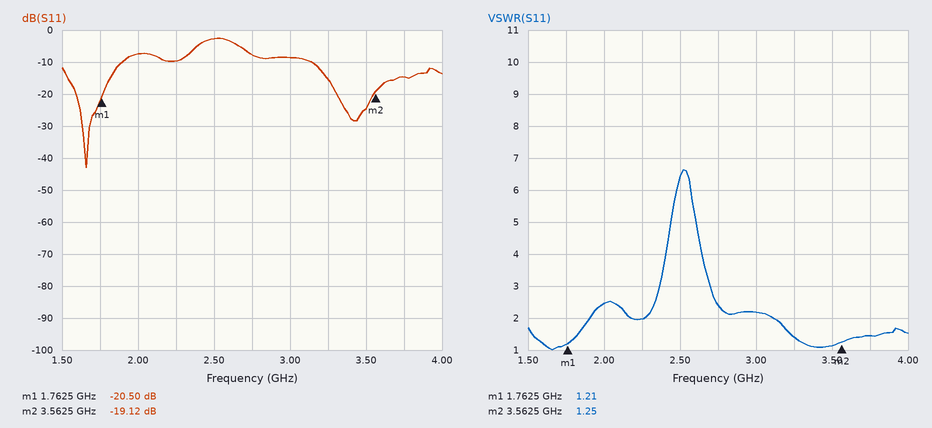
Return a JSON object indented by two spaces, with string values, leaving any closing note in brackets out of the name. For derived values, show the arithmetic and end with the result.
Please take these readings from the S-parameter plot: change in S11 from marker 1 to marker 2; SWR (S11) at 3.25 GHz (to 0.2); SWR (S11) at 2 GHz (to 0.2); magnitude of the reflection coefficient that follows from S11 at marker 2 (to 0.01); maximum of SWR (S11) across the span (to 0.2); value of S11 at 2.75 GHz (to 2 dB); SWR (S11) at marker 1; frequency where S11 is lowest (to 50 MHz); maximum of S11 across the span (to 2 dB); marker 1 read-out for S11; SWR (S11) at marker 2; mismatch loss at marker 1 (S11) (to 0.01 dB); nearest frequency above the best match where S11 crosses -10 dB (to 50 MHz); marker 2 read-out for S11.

{
  "change in S11 from marker 1 to marker 2": "-19.12 − (-20.5) = 1.38 dB",
  "SWR (S11) at 3.25 GHz": "1.4",
  "SWR (S11) at 2 GHz": "2.4",
  "magnitude of the reflection coefficient that follows from S11 at marker 2": "10^(-19.12/20) ≈ 0.11",
  "maximum of SWR (S11) across the span": "6.6",
  "value of S11 at 2.75 GHz": "-8 dB",
  "SWR (S11) at marker 1": "1.21",
  "frequency where S11 is lowest": "1.65 GHz",
  "maximum of S11 across the span": "-2 dB",
  "marker 1 read-out for S11": "-20.50 dB",
  "SWR (S11) at marker 2": "1.25",
  "mismatch loss at marker 1 (S11)": "−10 log10(1 − 10^(-20.5/10)) ≈ 0.04 dB",
  "nearest frequency above the best match where S11 crosses -10 dB": "1.90 GHz",
  "marker 2 read-out for S11": "-19.12 dB"
}
